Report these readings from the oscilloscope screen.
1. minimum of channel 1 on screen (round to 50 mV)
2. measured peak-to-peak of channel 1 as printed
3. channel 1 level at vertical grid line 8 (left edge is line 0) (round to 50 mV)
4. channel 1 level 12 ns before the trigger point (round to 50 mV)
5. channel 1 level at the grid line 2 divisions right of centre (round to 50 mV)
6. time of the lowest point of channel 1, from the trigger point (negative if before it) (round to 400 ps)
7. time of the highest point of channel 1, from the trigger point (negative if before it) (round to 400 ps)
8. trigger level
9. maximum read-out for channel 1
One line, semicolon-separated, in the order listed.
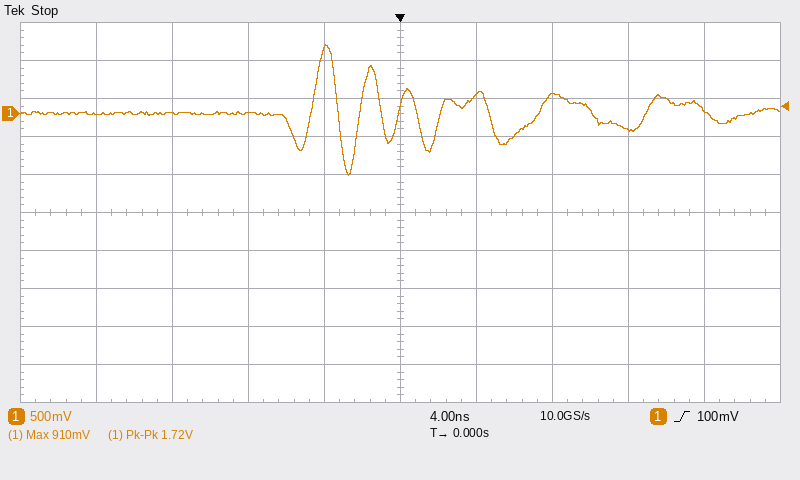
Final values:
-800 mV; 1.72 V; -200 mV; 0 mV; 250 mV; -2.8 ns; -4.0 ns; 100 mV; 910 mV
